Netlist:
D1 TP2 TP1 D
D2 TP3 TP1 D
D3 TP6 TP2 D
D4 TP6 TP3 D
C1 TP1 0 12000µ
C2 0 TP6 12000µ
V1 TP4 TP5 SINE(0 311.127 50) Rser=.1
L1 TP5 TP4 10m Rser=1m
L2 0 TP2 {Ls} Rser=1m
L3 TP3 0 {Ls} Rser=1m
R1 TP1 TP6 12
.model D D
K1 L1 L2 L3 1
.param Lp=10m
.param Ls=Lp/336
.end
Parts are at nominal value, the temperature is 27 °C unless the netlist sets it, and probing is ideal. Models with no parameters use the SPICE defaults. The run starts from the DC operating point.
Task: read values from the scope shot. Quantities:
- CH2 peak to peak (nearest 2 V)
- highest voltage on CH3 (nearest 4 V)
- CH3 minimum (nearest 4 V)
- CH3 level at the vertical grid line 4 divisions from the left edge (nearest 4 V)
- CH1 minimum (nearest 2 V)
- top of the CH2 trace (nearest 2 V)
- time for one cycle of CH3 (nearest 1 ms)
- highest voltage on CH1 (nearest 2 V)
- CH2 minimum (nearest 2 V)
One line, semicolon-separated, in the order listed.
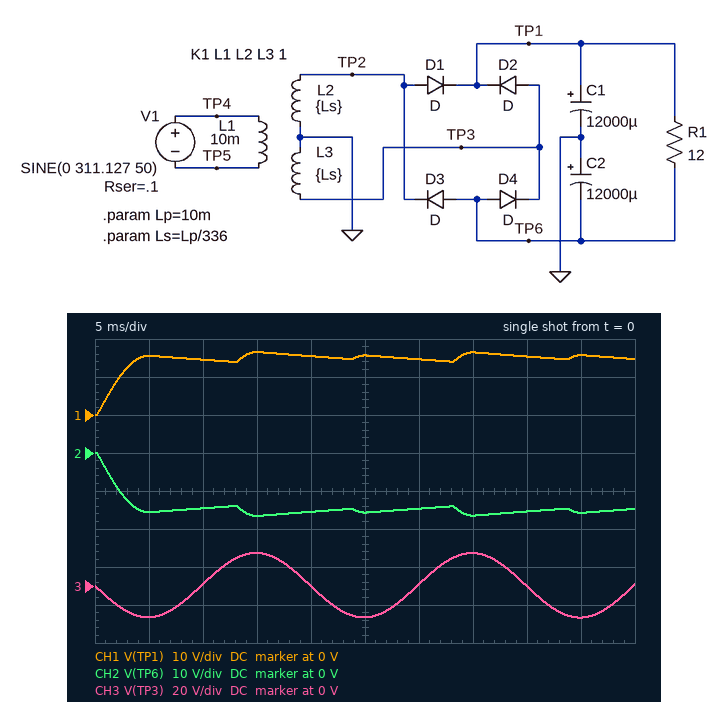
16 V; 16 V; -16 V; 0 V; 0 V; 0 V; 20 ms; 16 V; -16 V
